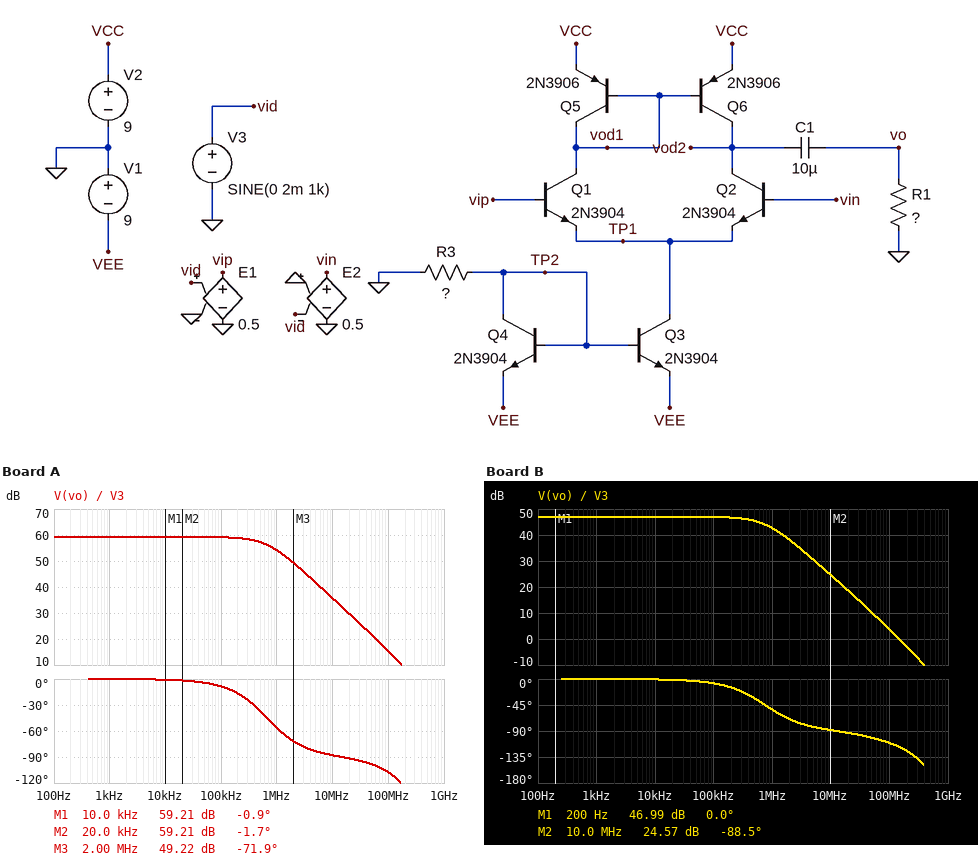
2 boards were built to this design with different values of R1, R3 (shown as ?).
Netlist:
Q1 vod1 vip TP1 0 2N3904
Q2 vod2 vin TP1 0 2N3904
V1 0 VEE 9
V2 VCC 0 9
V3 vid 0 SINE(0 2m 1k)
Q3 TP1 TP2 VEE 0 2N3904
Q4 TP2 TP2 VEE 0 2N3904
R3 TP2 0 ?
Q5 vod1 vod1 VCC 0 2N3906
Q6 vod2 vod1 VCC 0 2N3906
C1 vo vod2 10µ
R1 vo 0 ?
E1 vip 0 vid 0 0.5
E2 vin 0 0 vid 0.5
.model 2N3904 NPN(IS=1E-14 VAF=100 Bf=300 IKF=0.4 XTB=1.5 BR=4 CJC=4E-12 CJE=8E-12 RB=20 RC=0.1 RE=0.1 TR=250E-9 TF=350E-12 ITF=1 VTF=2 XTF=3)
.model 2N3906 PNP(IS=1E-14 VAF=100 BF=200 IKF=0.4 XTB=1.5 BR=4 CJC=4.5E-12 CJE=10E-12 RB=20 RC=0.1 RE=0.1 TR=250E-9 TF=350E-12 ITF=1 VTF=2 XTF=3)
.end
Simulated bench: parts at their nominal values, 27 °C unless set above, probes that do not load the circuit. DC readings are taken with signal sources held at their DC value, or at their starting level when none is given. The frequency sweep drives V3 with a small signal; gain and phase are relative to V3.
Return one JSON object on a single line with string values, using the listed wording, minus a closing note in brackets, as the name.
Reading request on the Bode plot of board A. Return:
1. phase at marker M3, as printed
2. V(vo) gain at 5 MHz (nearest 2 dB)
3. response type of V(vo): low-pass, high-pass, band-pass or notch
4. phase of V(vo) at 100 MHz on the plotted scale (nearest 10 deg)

{"phase at marker M3, as printed": "-71.9 deg", "V(vo) gain at 5 MHz": "42 dB", "response type of V(vo): low-pass, high-pass, band-pass or notch": "low-pass", "phase of V(vo) at 100 MHz on the plotted scale": "-110 deg"}
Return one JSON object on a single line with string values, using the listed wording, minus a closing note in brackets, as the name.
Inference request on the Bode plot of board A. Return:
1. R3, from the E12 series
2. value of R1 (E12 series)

{"R3, from the E12 series": "2.7 kΩ", "value of R1": "27 kΩ"}
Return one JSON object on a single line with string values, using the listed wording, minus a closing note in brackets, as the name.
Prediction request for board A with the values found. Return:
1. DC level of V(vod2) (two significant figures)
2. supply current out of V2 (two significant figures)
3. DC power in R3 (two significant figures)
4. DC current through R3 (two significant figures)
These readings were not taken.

{"DC level of V(vod2)": "7.8 V", "supply current out of V2": "3.3 mA", "DC power in R3": "26 mW", "DC current through R3": "3.1 mA"}
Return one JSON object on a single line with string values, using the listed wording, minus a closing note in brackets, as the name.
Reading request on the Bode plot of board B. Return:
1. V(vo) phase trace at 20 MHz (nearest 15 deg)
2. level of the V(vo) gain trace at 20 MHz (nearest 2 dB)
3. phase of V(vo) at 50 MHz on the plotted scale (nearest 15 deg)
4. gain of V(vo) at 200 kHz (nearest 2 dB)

{"V(vo) phase trace at 20 MHz": "-90 deg", "level of the V(vo) gain trace at 20 MHz": "18 dB", "phase of V(vo) at 50 MHz on the plotted scale": "-105 deg", "gain of V(vo) at 200 kHz": "46 dB"}
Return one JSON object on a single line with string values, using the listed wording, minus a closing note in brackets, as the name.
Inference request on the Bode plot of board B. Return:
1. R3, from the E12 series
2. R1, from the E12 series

{"R3, from the E12 series": "15 kΩ", "R1, from the E12 series": "22 kΩ"}
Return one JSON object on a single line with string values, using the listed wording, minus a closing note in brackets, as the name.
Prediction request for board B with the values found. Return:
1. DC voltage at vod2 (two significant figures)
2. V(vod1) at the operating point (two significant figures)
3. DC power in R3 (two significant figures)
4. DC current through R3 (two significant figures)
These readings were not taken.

{"DC voltage at vod2": "7.9 V", "V(vod1) at the operating point": "8.4 V", "DC power in R3": "4.7 mW", "DC current through R3": "560 µA"}
